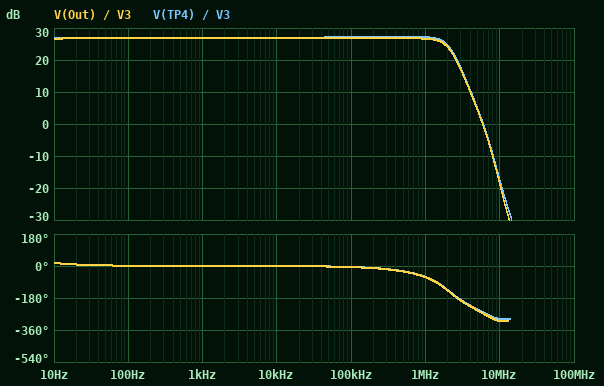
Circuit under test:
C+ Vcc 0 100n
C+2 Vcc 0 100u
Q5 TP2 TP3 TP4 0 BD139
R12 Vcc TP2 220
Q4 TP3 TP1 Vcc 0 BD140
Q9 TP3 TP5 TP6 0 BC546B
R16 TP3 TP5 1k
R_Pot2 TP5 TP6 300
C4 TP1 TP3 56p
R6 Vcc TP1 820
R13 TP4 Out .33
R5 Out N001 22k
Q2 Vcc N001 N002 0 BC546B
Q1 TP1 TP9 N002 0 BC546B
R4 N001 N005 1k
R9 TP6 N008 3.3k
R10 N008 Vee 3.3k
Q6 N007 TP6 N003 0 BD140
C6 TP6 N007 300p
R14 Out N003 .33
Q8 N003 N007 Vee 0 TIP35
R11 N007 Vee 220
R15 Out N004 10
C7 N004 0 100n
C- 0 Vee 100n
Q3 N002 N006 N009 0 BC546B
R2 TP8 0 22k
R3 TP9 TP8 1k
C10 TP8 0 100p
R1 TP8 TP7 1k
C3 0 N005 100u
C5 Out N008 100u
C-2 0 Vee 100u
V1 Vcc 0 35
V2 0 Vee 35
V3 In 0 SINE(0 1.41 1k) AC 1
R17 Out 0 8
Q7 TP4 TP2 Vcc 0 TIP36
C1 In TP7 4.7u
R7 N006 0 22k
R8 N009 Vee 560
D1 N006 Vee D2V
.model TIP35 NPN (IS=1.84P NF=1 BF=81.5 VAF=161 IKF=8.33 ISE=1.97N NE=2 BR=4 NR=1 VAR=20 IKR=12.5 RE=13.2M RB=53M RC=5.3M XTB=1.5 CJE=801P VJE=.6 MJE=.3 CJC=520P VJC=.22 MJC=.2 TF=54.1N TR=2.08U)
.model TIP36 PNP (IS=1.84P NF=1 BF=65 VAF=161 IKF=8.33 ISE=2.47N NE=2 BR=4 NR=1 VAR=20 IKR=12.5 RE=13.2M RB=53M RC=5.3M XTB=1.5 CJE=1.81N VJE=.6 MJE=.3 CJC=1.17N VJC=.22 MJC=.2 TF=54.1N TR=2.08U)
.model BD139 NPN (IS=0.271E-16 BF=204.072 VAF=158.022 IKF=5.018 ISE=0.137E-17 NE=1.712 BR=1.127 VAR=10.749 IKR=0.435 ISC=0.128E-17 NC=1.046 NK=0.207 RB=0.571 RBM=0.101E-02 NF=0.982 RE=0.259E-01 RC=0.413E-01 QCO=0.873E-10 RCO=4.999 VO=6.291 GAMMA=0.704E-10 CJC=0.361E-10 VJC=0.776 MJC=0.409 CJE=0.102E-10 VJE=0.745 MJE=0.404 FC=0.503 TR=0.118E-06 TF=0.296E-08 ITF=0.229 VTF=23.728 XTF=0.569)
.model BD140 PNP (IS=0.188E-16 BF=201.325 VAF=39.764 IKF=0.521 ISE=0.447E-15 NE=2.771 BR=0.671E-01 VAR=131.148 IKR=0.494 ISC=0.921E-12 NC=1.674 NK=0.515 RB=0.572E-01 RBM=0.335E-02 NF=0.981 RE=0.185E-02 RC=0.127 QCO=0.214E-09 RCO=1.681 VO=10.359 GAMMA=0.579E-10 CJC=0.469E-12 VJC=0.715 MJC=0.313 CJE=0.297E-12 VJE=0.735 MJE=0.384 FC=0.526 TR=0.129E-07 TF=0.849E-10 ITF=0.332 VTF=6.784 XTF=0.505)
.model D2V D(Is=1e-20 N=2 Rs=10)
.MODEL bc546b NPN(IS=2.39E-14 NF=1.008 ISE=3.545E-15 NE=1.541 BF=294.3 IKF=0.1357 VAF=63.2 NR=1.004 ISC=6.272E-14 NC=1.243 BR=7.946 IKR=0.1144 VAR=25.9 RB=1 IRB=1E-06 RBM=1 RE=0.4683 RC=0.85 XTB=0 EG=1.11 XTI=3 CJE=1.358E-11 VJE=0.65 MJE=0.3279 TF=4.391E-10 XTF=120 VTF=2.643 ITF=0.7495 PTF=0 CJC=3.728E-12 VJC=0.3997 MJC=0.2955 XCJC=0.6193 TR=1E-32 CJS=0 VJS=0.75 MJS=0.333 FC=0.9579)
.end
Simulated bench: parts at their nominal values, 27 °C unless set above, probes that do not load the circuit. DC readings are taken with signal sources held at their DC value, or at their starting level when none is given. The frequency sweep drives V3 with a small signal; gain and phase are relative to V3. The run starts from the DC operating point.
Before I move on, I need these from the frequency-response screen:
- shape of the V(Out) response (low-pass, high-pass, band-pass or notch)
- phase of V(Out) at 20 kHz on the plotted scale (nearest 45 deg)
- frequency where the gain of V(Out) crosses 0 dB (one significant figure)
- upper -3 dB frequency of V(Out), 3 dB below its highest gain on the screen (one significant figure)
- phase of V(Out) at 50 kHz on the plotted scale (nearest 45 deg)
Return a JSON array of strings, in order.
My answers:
["low-pass", "0 deg", "6 MHz", "2 MHz", "0 deg"]
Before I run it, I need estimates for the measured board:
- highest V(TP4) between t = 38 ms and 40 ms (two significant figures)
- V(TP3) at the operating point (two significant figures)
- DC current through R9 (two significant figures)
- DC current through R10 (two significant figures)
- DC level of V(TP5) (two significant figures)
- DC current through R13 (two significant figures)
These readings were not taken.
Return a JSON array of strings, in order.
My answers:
["32 V", "1.5 V", "5.1 mA", "5.1 mA", "-750 mV", "1.7 A"]
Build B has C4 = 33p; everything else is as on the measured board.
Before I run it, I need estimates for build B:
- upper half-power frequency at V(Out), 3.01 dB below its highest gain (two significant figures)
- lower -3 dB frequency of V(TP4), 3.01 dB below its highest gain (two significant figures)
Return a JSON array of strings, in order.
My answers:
["3.0 MHz", "2.4 Hz"]
